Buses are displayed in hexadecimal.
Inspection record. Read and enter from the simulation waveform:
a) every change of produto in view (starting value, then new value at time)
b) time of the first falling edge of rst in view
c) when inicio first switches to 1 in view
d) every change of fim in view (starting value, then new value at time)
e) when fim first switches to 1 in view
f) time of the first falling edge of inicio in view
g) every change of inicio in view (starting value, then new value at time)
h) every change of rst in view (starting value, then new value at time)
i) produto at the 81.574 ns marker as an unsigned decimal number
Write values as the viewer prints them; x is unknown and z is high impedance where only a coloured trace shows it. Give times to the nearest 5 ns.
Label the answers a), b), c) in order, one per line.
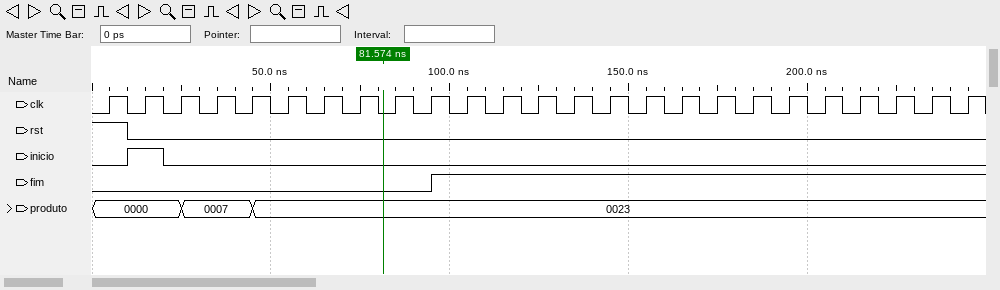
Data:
a) 0000, 0007 at 25 ns, 0023 at 45 ns
b) 10 ns
c) 10 ns
d) 0, 1 at 95 ns
e) 95 ns
f) 20 ns
g) 0, 1 at 10 ns, 0 at 20 ns
h) 1, 0 at 10 ns
i) 35
